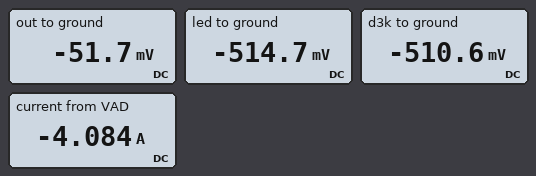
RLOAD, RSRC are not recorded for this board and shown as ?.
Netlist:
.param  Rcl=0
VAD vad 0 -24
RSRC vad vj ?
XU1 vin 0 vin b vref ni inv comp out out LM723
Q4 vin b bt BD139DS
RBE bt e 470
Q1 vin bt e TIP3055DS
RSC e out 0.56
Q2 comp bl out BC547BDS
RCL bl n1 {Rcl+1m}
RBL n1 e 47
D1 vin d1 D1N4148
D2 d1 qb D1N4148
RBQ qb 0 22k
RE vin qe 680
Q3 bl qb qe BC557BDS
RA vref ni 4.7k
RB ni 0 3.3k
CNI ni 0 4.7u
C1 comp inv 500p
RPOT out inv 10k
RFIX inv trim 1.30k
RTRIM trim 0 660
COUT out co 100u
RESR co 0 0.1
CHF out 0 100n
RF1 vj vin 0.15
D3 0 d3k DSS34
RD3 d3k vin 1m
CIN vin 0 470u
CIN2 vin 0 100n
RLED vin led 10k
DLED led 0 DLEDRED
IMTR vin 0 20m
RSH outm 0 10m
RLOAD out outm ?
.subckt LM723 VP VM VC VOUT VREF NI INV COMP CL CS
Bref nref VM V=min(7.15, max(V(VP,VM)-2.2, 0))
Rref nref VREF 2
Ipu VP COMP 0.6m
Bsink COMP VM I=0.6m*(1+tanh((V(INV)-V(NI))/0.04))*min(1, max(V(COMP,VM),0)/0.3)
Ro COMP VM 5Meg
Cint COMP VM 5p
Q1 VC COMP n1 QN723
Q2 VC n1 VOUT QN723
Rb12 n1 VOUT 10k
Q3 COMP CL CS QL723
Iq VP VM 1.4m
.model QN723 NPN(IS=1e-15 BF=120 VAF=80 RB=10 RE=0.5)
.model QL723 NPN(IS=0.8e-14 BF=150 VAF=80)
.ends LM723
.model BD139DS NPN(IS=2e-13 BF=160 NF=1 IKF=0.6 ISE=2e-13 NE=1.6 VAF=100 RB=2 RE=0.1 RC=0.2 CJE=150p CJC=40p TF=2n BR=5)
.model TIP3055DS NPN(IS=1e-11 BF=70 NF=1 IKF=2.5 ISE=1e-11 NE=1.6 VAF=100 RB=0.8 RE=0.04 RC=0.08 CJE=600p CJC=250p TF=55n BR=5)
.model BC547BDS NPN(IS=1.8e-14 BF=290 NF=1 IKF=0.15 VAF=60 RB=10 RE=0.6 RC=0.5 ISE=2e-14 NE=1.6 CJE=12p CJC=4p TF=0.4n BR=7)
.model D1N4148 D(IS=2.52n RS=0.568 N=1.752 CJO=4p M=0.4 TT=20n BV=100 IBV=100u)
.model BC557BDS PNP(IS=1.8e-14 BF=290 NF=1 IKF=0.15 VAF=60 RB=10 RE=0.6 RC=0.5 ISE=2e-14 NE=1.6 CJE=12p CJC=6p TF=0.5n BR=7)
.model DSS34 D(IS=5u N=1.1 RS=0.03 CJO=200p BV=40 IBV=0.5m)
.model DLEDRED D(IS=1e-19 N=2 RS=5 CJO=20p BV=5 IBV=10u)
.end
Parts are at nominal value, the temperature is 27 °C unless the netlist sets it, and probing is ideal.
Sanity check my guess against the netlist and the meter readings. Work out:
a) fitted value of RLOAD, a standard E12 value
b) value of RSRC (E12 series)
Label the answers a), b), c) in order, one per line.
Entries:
a) 180 Ω
b) 5.6 Ω
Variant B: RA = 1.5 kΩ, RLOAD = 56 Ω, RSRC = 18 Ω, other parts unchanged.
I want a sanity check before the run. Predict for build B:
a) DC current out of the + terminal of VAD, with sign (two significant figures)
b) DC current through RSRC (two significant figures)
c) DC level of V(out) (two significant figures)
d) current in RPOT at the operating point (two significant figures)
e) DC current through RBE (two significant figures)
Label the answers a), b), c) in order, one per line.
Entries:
a) -1.3 A
b) 1.3 A
c) -2.4 mV
d) 200 nA
e) 7.2 µA
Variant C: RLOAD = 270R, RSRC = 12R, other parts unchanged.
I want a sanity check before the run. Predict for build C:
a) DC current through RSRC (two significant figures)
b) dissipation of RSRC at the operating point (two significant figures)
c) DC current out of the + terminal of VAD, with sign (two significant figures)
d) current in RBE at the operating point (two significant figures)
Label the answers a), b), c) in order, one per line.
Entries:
a) 1.9 A
b) 45 W
c) -1.9 A
d) 12 µA
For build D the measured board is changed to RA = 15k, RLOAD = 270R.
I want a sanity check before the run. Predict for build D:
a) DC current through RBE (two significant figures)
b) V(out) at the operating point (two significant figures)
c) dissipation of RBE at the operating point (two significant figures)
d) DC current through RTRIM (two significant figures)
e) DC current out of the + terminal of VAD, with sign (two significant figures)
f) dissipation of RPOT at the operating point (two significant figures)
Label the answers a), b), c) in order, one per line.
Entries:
a) 39 µA
b) -62 mV
c) 720 nW
d) 5.2 µA
e) -4.1 A
f) 270 nW
